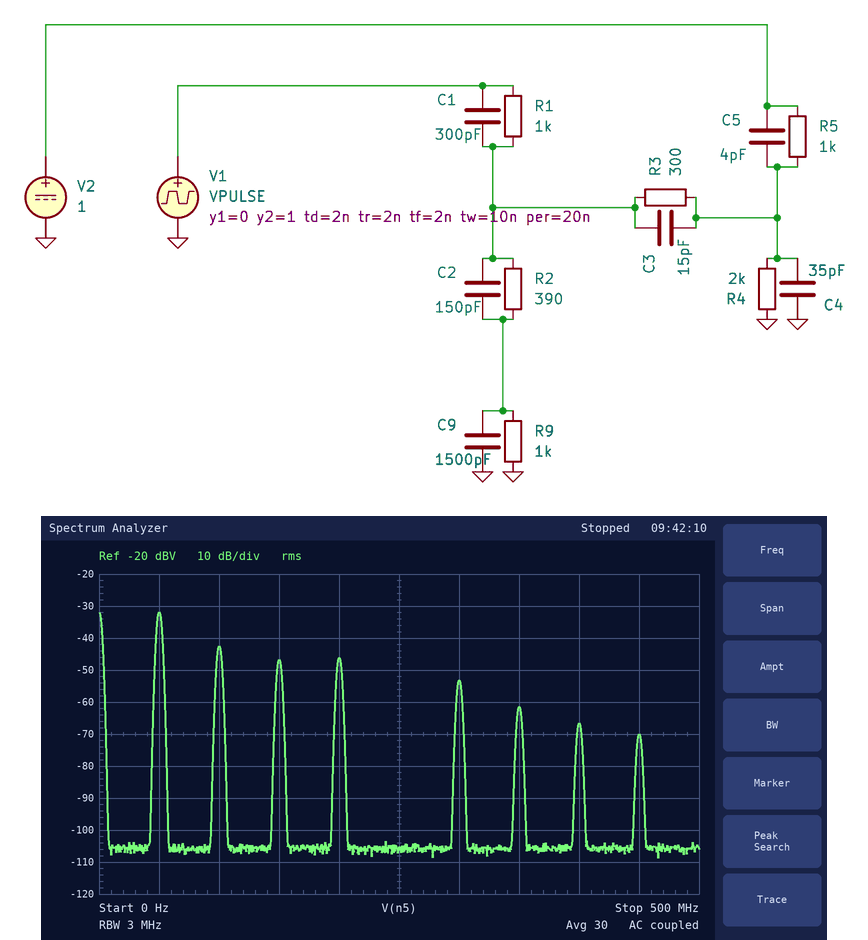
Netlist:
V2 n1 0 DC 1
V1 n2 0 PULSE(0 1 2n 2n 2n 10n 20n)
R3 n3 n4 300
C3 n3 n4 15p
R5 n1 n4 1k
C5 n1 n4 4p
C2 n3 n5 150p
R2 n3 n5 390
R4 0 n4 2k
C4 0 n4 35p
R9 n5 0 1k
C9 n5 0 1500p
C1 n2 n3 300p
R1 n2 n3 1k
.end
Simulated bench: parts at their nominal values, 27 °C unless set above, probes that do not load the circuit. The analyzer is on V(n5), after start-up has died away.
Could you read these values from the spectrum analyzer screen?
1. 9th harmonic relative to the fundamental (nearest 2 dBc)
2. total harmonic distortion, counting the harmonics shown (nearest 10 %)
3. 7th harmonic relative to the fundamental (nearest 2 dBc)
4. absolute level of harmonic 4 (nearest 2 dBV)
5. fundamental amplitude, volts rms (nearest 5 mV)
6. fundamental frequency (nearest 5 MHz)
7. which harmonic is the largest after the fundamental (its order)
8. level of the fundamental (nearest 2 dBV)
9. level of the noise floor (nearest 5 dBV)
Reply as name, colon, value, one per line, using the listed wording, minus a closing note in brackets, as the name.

9th harmonic relative to the fundamental: -38 dBc
total harmonic distortion, counting the harmonics shown: 40 %
7th harmonic relative to the fundamental: -30 dBc
absolute level of harmonic 4: -46 dBV
fundamental amplitude, volts rms: 25 mV
fundamental frequency: 50 MHz
which harmonic is the largest after the fundamental: 2
level of the fundamental: -32 dBV
level of the noise floor: -105 dBV
